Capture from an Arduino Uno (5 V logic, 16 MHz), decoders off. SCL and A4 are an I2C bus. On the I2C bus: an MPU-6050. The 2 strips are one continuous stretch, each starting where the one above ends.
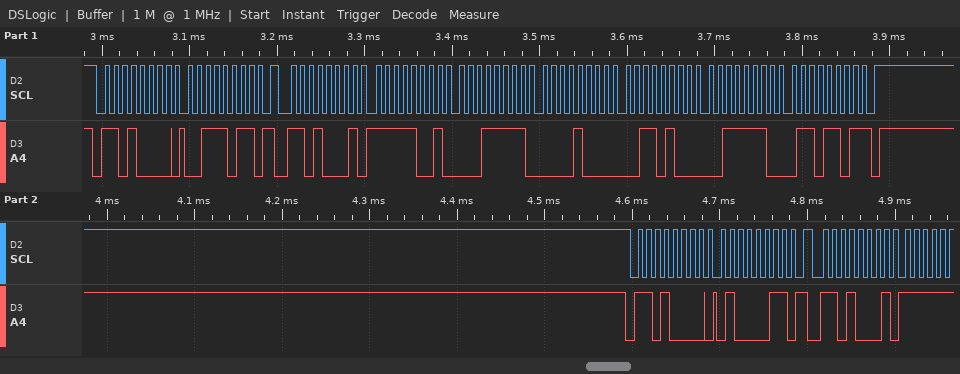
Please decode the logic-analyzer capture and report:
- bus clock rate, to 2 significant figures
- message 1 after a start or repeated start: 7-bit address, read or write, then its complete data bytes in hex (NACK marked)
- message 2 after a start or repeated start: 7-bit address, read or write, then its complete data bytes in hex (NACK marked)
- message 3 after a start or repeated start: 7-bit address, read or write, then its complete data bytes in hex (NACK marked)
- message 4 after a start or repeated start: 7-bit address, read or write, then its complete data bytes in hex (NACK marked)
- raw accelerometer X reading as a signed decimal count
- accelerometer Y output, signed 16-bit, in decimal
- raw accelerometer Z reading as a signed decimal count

100 kHz
0x68 write: 3B
0x68 read: F9 1F 08 34 3E 6D NACK
0x68 write: 43
0x68 read
-1761
2100
15981
